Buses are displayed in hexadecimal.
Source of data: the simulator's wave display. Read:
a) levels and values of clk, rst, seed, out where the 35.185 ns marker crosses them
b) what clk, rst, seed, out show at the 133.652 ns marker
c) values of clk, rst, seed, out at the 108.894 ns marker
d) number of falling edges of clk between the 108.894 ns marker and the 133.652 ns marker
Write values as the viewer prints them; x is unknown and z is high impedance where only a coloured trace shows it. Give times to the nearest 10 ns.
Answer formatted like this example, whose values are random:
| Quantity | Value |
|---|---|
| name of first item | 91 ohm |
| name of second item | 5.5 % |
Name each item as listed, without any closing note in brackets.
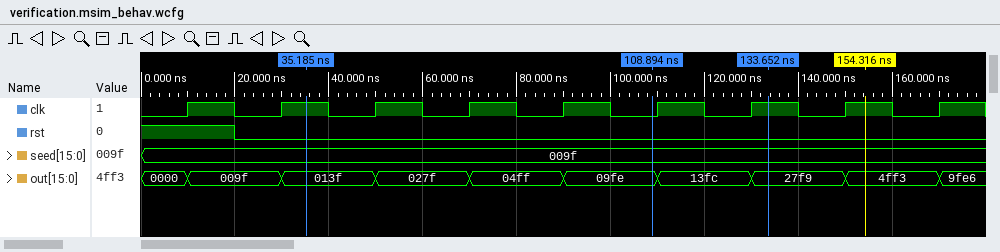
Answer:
| Quantity | Value |
|---|---|
| levels and values of clk, rst, seed, out where the 35.185 ns marker crosses them | clk=1, rst=0, seed=009f, out=013f |
| what clk, rst, seed, out show at the 133.652 ns marker | clk=1, rst=0, seed=009f, out=27f9 |
| values of clk, rst, seed, out at the 108.894 ns marker | clk=0, rst=0, seed=009f, out=09fe |
| number of falling edges of clk between the 108.894 ns marker and the 133.652 ns marker | 1 |
